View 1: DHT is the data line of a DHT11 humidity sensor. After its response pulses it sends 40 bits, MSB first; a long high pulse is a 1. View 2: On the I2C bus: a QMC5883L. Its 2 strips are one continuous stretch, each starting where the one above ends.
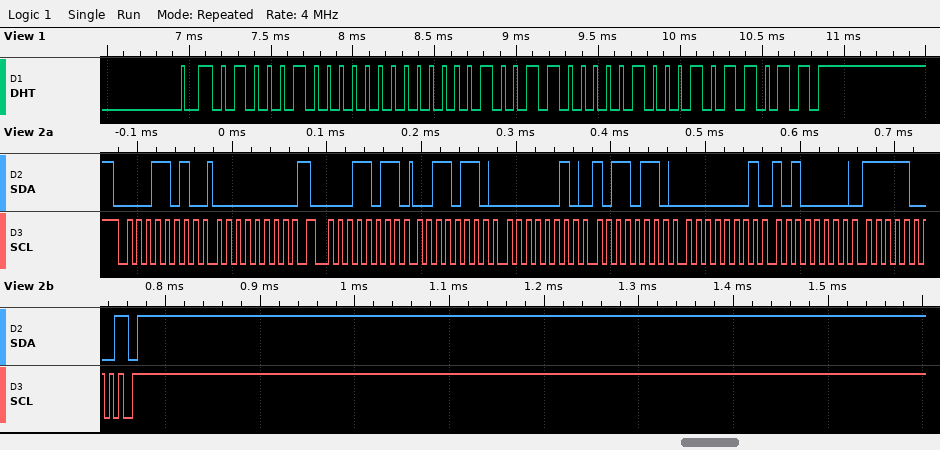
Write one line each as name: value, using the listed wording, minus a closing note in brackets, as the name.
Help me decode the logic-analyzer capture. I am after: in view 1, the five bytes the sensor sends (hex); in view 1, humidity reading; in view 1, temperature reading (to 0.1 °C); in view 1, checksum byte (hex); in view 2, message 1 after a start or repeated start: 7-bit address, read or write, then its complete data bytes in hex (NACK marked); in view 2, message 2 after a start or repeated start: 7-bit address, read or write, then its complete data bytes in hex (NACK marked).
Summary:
in view 1, the five bytes the sensor sends: 44 00 13 04 5B
in view 1, humidity reading: 68 %
in view 1, temperature reading: 19.4 °C
in view 1, checksum byte: 0x5B
in view 2, message 1 after a start or repeated start: 7-bit address, read or write, then its complete data bytes in hex: 0x0D write: 00
in view 2, message 2 after a start or repeated start: 7-bit address, read or write, then its complete data bytes in hex: 0x0D read: 36 02 B6 01 A0 F8 NACK
